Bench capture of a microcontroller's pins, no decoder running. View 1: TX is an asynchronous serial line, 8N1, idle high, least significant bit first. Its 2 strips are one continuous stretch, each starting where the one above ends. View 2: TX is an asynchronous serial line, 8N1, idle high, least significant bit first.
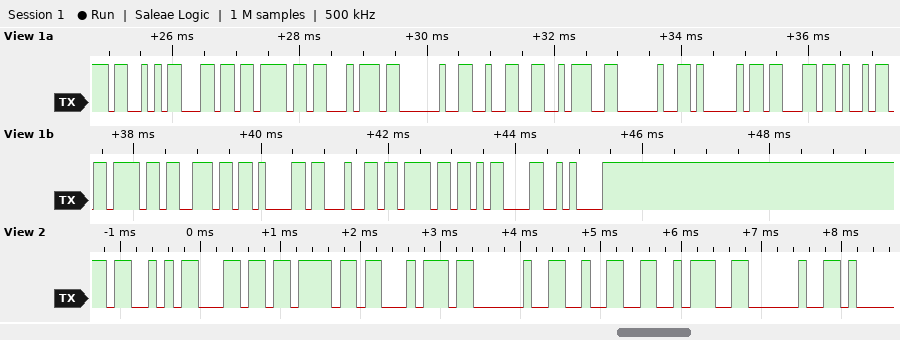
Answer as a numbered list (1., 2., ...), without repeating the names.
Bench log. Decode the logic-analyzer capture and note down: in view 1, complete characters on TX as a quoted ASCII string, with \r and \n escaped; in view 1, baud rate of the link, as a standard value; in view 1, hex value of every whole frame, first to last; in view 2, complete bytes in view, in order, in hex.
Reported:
1. "Slot 2: Acionado\r\n"
2. 9600 baud
3. 53 6C 6F 74 20 32 3A 20 41 63 69 6F 6E 61 64 6F 0D 0A
4. 53 6C 6F 74 20 32 3A 20
